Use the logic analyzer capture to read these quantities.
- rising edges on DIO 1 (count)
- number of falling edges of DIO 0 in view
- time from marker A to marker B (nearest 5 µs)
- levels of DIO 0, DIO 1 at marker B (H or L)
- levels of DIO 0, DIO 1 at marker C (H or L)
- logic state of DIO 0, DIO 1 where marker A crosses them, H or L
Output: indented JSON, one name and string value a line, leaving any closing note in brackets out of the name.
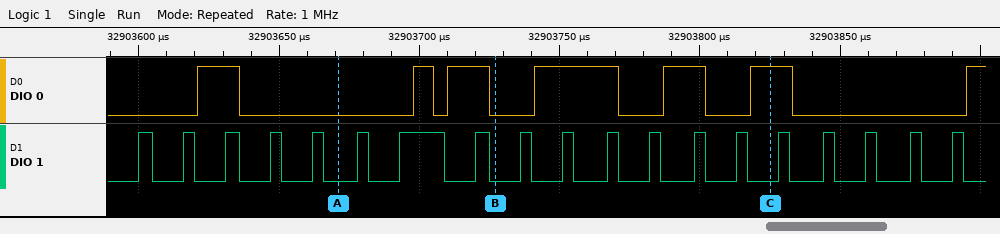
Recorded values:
{
  "rising edges on DIO 1": "19",
  "number of falling edges of DIO 0 in view": "6",
  "time from marker A to marker B": "55 µs",
  "levels of DIO 0, DIO 1 at marker B": "DIO 0=L, DIO 1=L",
  "levels of DIO 0, DIO 1 at marker C": "DIO 0=H, DIO 1=L",
  "logic state of DIO 0, DIO 1 where marker A crosses them, H or L": "DIO 0=L, DIO 1=L"
}
